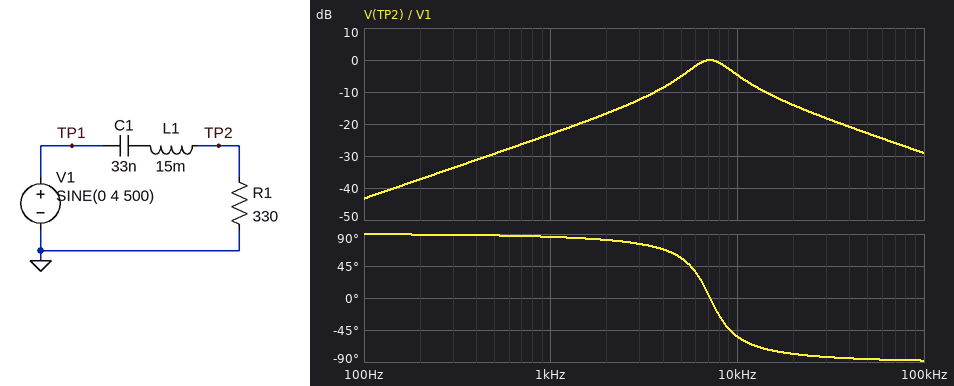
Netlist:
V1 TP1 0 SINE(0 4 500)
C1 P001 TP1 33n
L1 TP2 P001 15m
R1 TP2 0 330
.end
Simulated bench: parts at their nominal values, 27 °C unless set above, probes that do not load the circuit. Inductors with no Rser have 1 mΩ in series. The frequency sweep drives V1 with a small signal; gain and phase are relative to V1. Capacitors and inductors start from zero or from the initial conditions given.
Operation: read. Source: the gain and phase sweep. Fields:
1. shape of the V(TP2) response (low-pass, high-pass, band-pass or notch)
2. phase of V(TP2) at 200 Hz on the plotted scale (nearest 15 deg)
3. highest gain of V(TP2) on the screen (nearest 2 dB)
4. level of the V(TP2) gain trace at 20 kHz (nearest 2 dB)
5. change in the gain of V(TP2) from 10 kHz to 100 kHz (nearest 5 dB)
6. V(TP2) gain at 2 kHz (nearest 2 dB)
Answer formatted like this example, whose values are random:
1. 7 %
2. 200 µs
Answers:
1. band-pass
2. 90 deg
3. 0 dB
4. -14 dB
5. -25 dB
6. -16 dB
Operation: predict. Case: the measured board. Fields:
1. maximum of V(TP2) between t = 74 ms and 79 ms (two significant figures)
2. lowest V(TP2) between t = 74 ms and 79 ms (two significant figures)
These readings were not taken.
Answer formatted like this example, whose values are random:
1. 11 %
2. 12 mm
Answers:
1. 140 mV
2. -140 mV
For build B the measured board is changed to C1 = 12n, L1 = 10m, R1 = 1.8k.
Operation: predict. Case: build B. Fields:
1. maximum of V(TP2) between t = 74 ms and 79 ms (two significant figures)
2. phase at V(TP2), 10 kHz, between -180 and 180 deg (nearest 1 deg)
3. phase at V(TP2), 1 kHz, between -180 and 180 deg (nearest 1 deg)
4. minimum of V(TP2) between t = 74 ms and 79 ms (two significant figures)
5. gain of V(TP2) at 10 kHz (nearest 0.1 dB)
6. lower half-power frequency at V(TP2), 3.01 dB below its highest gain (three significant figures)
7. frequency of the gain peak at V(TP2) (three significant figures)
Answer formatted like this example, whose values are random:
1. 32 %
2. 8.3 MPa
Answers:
1. 270 mV
2. 21 deg
3. 82 deg
4. -270 mV
5. -0.6 dB
6. 6.08 kHz
7. 14.5 kHz
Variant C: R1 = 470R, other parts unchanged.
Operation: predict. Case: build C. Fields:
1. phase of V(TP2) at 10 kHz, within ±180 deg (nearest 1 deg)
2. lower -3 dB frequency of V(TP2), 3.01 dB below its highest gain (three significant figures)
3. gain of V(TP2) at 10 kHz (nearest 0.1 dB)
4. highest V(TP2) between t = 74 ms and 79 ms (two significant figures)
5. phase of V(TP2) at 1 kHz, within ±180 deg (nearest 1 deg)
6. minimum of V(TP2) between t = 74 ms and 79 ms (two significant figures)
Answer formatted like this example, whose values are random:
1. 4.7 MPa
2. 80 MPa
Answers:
1. -44 deg
2. 5.08 kHz
3. -2.9 dB
4. 200 mV
5. 84 deg
6. -200 mV
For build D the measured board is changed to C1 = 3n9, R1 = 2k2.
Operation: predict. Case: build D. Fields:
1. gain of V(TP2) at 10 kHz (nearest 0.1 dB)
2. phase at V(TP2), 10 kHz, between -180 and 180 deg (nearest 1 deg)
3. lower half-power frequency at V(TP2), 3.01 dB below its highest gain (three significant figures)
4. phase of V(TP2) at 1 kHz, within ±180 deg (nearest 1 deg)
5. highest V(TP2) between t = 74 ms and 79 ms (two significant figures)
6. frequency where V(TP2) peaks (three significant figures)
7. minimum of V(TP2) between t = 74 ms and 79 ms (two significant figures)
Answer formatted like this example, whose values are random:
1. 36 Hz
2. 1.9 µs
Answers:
1. -4.8 dB
2. 55 deg
3. 12.2 kHz
4. 87 deg
5. 110 mV
6. 20.8 kHz
7. -110 mV
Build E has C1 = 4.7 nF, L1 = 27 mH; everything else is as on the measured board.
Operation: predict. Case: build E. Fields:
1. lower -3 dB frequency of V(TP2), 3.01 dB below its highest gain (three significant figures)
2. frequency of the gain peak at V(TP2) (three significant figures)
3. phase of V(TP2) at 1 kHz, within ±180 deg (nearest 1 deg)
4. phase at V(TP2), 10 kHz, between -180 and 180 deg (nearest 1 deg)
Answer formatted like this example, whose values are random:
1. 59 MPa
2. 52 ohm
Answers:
1. 13.2 kHz
2. 14.1 kHz
3. 89 deg
4. 79 deg
